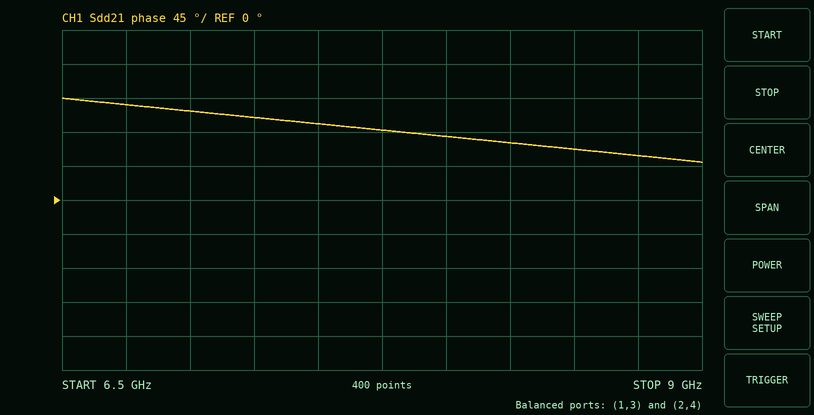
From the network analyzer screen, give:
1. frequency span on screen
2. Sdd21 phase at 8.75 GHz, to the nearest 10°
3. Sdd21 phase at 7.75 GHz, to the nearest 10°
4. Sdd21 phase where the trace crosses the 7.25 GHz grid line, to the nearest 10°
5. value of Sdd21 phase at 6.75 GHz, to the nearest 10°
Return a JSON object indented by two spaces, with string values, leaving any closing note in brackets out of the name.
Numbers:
{
  "frequency span on screen": "2.5 GHz",
  "Sdd21 phase at 8.75 GHz, to the nearest 10°": "60°",
  "Sdd21 phase at 7.75 GHz, to the nearest 10°": "90°",
  "Sdd21 phase where the trace crosses the 7.25 GHz grid line, to the nearest 10°": "110°",
  "value of Sdd21 phase at 6.75 GHz, to the nearest 10°": "130°"
}
